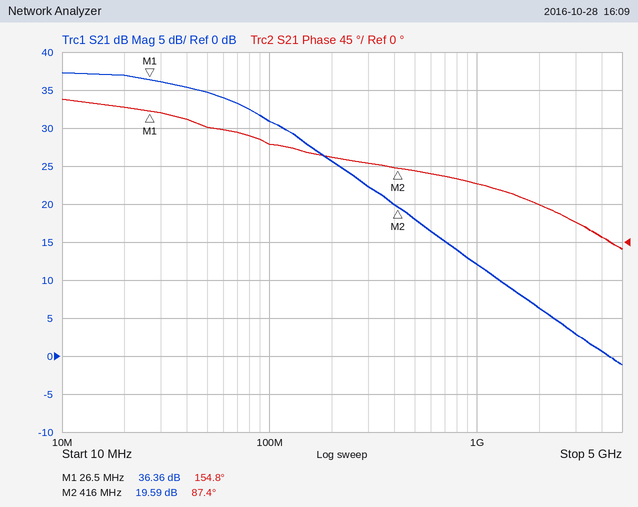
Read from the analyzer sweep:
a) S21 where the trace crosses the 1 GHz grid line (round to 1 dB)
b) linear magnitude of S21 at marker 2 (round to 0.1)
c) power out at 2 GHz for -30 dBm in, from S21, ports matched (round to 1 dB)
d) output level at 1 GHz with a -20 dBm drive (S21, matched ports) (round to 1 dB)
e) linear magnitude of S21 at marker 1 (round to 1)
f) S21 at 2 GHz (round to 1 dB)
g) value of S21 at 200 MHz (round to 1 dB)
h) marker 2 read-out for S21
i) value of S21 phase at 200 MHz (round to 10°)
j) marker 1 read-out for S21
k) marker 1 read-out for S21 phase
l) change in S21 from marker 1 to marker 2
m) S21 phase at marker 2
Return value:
12 dB
9.5
-24 dBm
-8 dBm
66
6 dB
26 dB
19.59 dB
100°
36.36 dB
154.8°
-16.77 dB
87.4°
